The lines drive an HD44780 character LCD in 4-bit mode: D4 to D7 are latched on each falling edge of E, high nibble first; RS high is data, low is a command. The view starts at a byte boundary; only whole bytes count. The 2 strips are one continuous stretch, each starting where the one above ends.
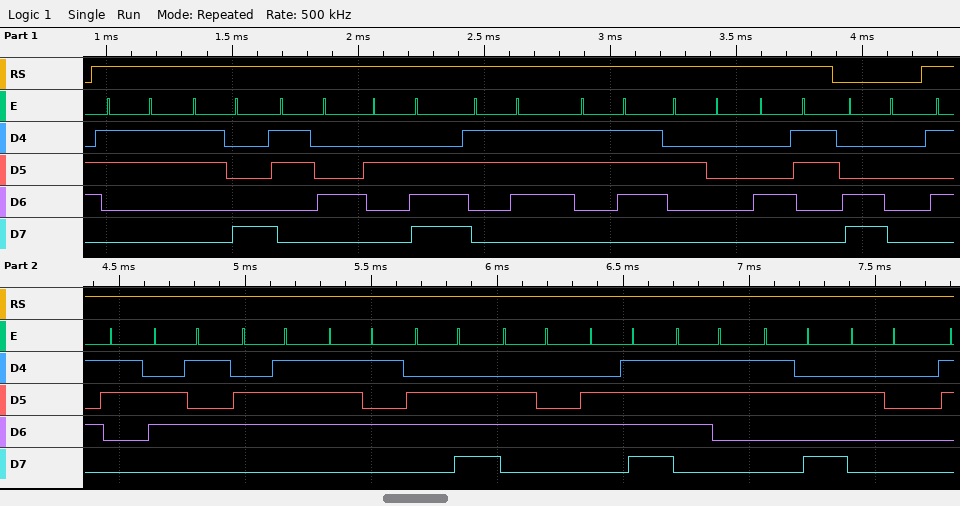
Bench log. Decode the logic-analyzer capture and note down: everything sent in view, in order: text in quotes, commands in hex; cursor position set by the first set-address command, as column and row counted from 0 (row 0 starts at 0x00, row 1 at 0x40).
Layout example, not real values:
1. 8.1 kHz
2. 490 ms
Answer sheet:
1. "384.77 C" 0xC0 "Segundos: "
2. column 0, row 1
